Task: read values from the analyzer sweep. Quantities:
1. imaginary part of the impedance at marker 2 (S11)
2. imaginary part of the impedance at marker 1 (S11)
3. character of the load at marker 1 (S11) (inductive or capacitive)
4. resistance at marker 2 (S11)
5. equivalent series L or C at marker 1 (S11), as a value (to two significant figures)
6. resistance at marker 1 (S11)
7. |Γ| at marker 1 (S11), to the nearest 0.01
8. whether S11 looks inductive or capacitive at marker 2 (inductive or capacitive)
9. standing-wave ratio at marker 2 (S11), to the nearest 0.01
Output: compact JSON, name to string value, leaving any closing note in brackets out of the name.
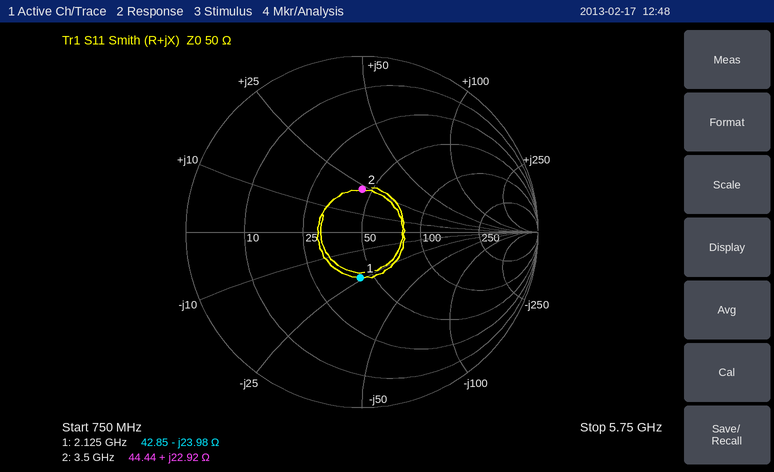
{"imaginary part of the impedance at marker 2": "+22.92 Ω", "imaginary part of the impedance at marker 1": "-23.98 Ω", "character of the load at marker 1 (S11)": "capacitive", "resistance at marker 2": "44.44 Ω", "equivalent series L or C at marker 1 (S11), as a value": "3.1 pF", "resistance at marker 1": "42.85 Ω", "|Γ| at marker 1 (S11), to the nearest 0.01": "0.26", "whether S11 looks inductive or capacitive at marker 2": "inductive", "standing-wave ratio at marker 2 (S11), to the nearest 0.01": "1.64"}
